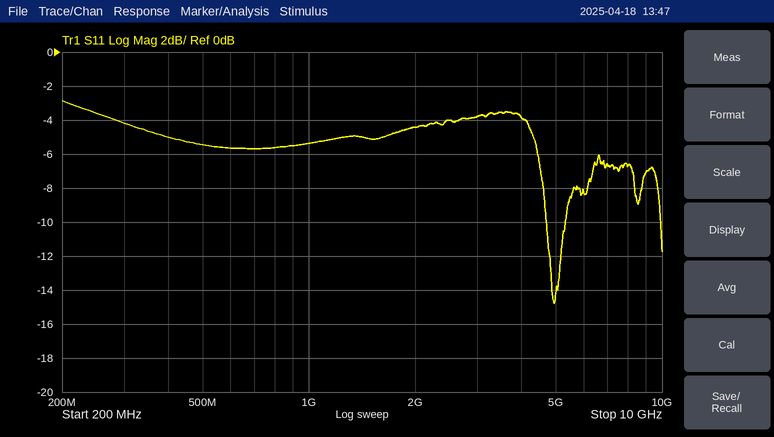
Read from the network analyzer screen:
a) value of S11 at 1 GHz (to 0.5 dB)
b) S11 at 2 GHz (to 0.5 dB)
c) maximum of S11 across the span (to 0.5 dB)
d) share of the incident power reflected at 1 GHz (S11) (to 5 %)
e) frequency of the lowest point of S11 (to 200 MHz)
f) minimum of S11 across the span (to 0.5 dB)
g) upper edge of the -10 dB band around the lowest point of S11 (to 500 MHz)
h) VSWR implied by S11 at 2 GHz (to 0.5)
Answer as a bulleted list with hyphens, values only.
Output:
- -5.5 dB
- -4.5 dB
- -3.0 dB
- 30 %
- 5.0 GHz
- -15.0 dB
- 5.5 GHz
- 4.0
